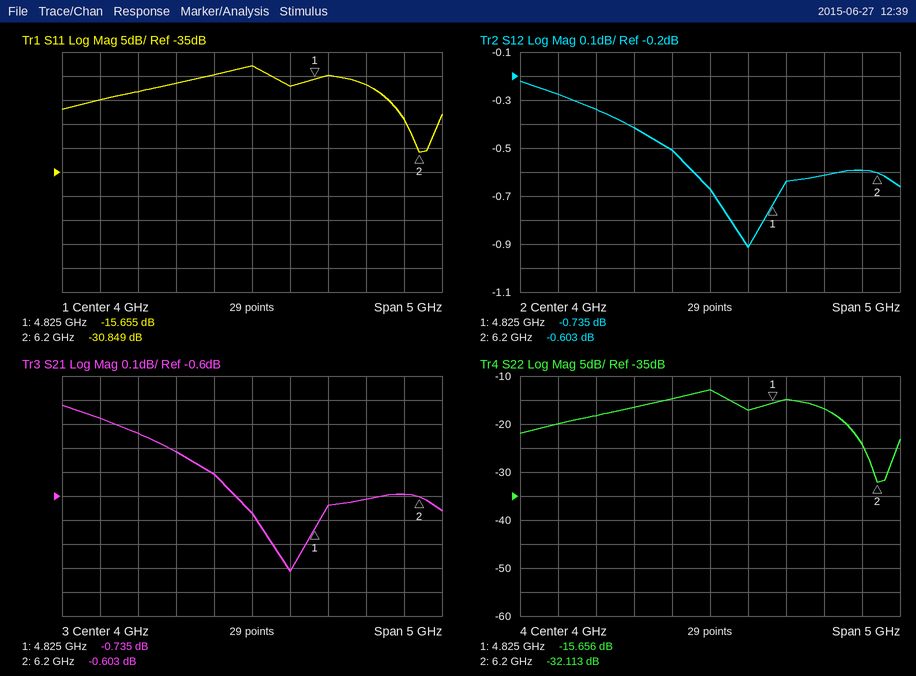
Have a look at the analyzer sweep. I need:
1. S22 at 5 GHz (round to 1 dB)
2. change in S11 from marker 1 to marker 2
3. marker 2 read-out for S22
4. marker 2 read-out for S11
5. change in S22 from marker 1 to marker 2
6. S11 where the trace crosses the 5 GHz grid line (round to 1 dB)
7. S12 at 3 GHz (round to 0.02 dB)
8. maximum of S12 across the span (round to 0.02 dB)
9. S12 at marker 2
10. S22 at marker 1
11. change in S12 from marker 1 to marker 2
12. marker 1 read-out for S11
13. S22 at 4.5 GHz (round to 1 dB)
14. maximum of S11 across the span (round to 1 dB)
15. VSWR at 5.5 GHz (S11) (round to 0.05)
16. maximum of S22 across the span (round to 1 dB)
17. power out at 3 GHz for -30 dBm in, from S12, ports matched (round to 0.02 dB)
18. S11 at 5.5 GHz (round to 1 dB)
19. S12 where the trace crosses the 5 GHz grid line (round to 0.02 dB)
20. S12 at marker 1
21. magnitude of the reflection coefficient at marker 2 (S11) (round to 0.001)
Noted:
-15 dB
-15.194 dB
-32.113 dB
-30.849 dB
-16.457 dB
-15 dB
-0.42 dB
-0.22 dB
-0.603 dB
-15.656 dB
0.132 dB
-15.655 dB
-17 dB
-13 dB
1.35
-13 dB
-30.42 dBm
-17 dB
-0.64 dB
-0.735 dB
0.029
